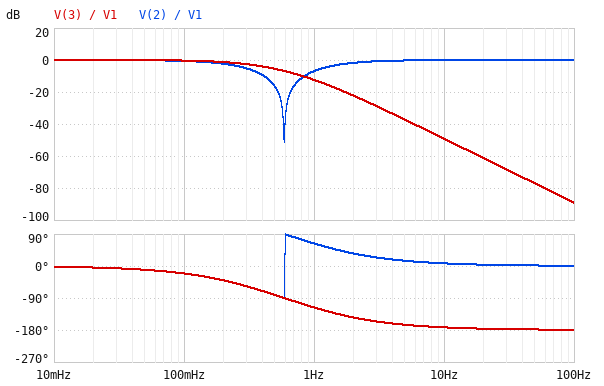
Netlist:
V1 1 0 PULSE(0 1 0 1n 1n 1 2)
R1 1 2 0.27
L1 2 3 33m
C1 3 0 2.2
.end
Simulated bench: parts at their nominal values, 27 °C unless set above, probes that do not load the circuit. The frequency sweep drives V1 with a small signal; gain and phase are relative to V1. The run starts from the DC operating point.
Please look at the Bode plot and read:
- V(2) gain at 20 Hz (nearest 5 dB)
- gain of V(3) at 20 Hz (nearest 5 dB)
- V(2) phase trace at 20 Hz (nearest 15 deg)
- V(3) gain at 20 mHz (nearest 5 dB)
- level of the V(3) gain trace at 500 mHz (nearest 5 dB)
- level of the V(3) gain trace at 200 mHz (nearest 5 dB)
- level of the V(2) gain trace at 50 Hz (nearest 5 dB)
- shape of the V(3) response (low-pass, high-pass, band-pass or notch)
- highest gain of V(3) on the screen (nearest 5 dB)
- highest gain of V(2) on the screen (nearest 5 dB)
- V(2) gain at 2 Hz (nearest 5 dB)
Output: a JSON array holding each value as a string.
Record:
["0 dB", "-60 dB", "0 deg", "0 dB", "-5 dB", "0 dB", "0 dB", "low-pass", "0 dB", "0 dB", "0 dB"]
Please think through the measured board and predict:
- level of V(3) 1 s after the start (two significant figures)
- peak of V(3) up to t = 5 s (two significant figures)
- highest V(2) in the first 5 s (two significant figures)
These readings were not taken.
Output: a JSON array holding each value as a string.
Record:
["840 mV", "860 mV", "1.2 V"]
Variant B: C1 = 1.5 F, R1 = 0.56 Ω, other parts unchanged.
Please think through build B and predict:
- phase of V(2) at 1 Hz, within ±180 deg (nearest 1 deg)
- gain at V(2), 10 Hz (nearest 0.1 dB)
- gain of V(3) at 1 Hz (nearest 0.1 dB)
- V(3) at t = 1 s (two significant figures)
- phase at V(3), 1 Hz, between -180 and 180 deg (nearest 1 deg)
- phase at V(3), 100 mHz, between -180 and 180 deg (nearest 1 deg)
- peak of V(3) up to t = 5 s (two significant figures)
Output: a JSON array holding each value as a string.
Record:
["80 deg", "-0.3 dB", "-14.6 dB", "700 mV", "-100 deg", "-28 deg", "760 mV"]
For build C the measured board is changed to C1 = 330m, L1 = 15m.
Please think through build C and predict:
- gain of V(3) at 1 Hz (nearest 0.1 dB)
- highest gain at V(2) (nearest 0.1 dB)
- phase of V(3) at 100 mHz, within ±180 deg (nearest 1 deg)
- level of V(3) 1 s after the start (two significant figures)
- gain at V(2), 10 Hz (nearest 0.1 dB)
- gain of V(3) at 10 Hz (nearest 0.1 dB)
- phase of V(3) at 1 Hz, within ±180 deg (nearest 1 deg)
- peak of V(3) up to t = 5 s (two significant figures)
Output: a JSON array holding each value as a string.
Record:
["0.2 dB", "0 dB", "-3 deg", "1.0 V", "-0.4 dB", "-25.7 dB", "-35 deg", "1.1 V"]
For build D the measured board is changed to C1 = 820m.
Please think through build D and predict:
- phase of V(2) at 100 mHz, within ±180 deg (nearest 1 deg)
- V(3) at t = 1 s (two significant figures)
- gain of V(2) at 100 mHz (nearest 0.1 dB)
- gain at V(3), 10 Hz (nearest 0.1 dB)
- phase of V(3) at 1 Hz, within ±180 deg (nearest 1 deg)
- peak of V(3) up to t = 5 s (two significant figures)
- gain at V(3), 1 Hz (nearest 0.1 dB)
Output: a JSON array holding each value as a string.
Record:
["-8 deg", "1.0 V", "-0.1 dB", "-40.6 dB", "-93 deg", "1.1 V", "-2.9 dB"]
